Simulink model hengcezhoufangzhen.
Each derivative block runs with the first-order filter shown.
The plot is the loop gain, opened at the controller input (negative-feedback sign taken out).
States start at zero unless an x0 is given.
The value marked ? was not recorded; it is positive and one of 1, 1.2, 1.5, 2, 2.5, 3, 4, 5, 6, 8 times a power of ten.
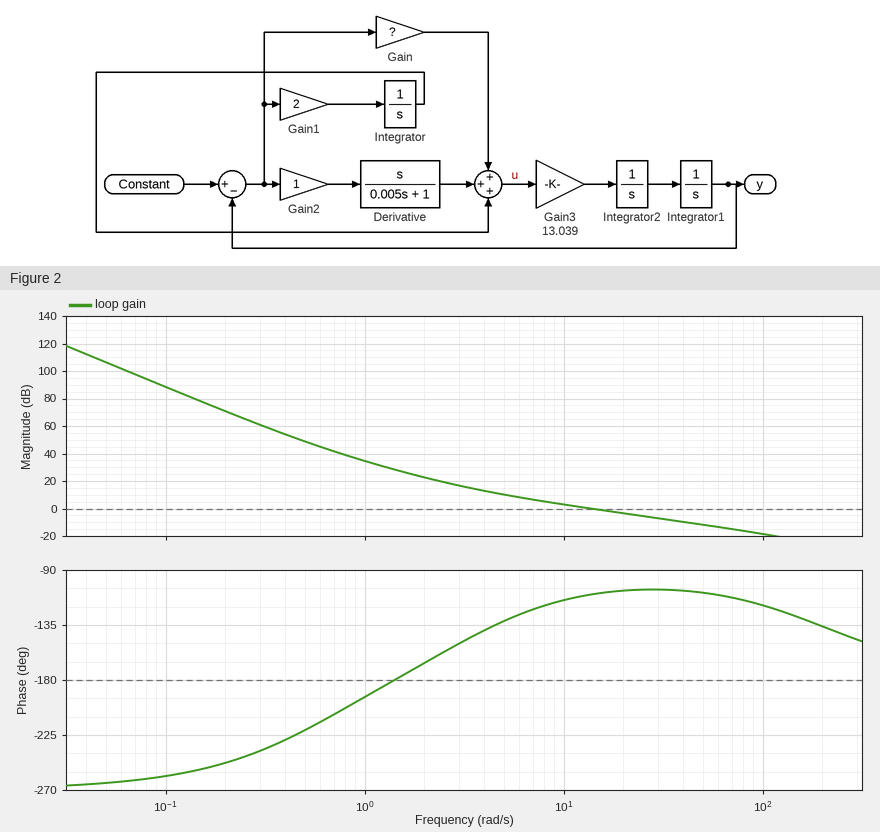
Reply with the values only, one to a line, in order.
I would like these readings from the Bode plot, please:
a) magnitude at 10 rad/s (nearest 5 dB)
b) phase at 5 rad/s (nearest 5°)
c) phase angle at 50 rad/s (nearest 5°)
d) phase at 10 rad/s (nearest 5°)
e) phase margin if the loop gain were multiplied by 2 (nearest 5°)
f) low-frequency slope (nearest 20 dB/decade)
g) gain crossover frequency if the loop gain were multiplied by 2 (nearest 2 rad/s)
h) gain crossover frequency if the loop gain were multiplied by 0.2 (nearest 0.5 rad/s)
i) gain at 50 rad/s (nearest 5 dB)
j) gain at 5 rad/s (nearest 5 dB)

5 dB
-130°
-110°
-115°
75°
-60 dB/decade
26 rad/s
3.5 rad/s
-10 dB
10 dB
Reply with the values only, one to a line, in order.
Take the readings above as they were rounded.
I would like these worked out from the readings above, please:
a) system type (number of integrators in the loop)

3
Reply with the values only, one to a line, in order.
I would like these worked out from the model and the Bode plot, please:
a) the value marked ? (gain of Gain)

4
